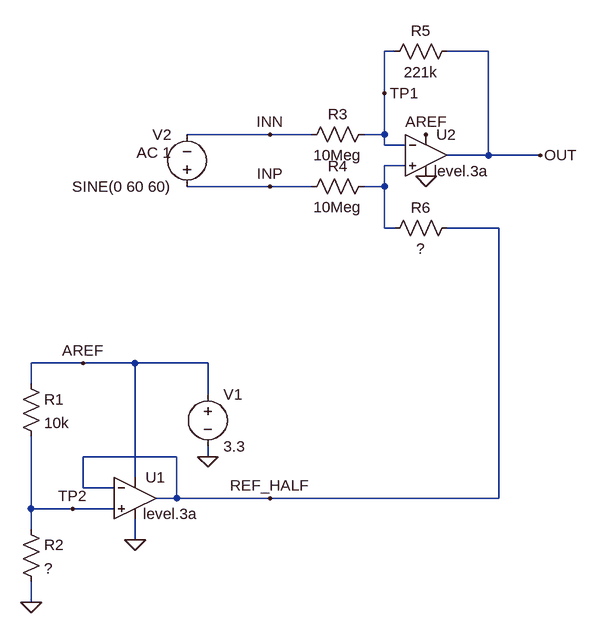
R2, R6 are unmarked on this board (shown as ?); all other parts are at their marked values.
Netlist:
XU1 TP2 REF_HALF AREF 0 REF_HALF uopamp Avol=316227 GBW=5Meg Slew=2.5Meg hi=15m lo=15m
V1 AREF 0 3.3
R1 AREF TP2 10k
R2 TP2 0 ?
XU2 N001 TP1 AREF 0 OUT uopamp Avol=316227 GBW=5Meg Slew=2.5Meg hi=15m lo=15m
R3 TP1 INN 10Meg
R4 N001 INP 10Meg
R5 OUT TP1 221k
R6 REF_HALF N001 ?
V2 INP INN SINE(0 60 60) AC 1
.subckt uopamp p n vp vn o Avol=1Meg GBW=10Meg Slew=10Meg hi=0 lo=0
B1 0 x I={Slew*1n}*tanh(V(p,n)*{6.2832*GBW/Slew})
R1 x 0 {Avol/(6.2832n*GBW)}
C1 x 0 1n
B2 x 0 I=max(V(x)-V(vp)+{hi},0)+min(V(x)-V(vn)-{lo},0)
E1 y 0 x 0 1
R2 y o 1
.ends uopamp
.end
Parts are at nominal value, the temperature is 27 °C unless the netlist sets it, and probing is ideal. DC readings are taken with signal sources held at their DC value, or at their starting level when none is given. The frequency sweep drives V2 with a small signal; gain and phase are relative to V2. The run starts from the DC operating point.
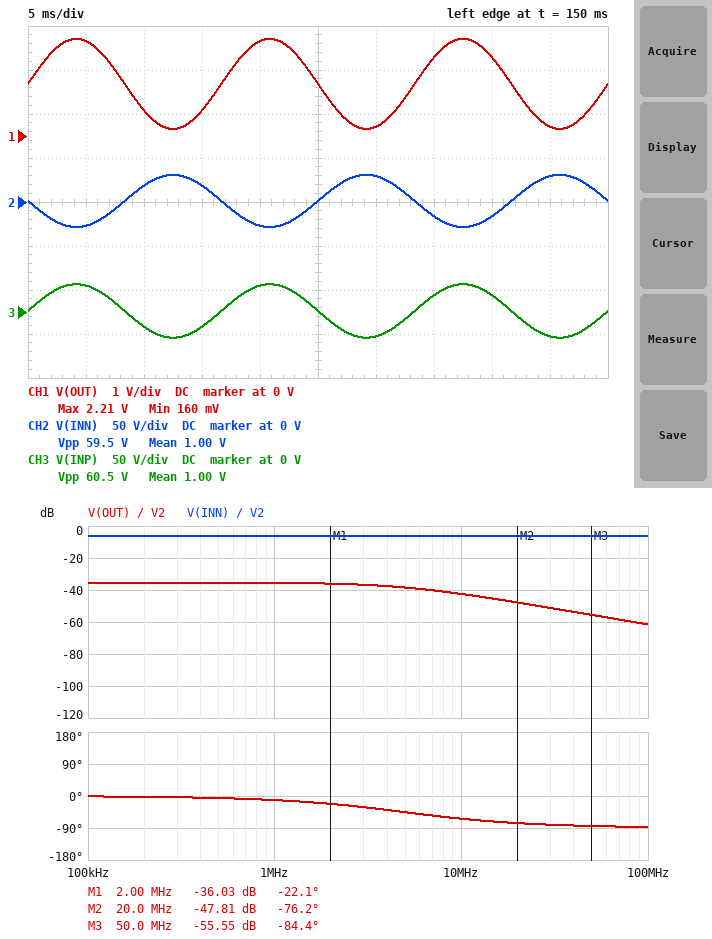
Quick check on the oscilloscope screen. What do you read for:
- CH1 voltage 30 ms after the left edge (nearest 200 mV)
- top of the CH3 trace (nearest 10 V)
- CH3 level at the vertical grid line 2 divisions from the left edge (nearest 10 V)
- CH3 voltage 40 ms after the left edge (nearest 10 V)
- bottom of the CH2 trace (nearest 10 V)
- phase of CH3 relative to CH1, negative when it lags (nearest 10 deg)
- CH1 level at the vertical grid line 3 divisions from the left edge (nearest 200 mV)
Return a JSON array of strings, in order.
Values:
["200 mV", "30 V", "-20 V", "20 V", "-30 V", "0 deg", "600 mV"]
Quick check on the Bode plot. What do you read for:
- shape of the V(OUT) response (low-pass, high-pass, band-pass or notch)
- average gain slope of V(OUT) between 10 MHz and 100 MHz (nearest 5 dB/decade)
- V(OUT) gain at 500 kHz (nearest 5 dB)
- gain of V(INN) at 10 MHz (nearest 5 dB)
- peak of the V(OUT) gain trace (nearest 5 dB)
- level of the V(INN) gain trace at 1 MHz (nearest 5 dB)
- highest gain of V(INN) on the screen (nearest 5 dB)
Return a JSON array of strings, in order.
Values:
["low-pass", "-20 dB/decade", "-35 dB", "-5 dB", "-35 dB", "-5 dB", "-5 dB"]
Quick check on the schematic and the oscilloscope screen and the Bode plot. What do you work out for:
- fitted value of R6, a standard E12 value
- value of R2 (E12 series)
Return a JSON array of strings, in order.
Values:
["120 kΩ", "5.6 kΩ"]
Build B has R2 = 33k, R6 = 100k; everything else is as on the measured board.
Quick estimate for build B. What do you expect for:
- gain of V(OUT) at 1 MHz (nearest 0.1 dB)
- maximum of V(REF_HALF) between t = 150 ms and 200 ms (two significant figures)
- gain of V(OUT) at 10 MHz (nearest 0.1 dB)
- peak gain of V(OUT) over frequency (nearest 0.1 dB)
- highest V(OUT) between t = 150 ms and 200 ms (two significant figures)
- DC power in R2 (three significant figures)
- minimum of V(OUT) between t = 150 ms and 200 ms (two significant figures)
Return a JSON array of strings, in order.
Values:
["-36.1 dB", "2.5 V", "-43.0 dB", "-35.9 dB", "3.3 V", "194 µW", "1.6 V"]
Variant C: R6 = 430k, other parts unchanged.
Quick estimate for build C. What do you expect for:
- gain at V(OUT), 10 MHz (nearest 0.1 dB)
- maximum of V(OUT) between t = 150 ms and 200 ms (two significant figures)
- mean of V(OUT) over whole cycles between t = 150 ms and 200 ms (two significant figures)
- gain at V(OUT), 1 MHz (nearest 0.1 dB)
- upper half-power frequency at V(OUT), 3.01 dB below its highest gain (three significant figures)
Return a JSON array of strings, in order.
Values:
["-37.0 dB", "3.1 V", "1.3 V", "-29.9 dB", "4.84 MHz"]
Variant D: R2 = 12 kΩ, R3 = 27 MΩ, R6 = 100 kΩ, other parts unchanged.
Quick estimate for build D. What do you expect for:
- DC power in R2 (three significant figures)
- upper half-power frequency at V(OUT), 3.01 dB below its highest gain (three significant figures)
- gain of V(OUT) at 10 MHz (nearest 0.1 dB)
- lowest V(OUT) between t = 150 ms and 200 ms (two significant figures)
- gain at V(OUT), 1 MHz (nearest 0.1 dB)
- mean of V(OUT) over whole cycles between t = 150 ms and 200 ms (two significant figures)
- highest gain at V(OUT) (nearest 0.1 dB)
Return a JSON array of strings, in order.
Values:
["270 µW", "4.96 MHz", "-48.3 dB", "1.3 V", "-41.4 dB", "1.8 V", "-41.2 dB"]
